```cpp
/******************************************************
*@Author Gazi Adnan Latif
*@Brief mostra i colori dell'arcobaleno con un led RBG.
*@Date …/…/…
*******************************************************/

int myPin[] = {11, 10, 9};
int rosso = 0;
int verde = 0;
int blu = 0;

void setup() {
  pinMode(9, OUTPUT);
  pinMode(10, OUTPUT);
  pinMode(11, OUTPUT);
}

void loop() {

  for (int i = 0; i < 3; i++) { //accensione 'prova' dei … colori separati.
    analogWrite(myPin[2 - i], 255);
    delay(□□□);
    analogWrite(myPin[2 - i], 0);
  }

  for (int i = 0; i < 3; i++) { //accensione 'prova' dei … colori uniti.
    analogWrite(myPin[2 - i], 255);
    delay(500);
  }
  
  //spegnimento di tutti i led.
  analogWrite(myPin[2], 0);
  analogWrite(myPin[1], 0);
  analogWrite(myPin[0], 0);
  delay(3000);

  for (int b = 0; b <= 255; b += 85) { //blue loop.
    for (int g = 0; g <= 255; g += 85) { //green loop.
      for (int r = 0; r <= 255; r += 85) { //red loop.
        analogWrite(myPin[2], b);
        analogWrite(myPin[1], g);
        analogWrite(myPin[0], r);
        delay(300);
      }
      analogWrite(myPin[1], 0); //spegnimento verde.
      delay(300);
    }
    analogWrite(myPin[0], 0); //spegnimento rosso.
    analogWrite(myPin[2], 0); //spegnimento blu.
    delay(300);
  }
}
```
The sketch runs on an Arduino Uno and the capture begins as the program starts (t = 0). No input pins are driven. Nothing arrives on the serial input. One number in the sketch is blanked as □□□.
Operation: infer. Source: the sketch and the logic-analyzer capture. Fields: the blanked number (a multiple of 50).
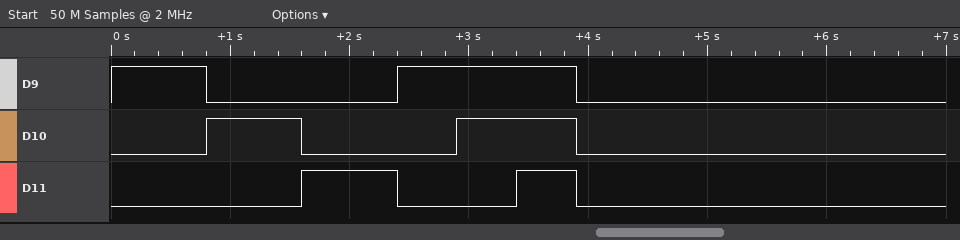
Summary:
800
